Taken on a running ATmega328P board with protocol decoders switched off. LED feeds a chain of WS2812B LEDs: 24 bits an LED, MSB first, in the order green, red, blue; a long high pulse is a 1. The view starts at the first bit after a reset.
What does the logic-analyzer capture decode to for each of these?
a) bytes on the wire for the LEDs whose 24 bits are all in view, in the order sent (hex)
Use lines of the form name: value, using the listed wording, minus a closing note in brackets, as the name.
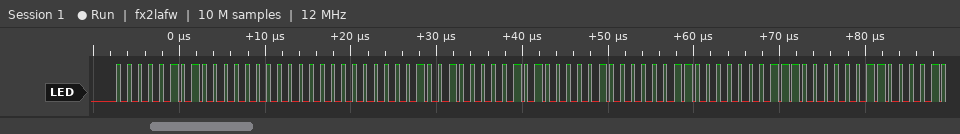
bytes on the wire for the LEDs whose 24 bits are all in view, in the order sent: 05 00 00 09 05 04 0C 07 03
